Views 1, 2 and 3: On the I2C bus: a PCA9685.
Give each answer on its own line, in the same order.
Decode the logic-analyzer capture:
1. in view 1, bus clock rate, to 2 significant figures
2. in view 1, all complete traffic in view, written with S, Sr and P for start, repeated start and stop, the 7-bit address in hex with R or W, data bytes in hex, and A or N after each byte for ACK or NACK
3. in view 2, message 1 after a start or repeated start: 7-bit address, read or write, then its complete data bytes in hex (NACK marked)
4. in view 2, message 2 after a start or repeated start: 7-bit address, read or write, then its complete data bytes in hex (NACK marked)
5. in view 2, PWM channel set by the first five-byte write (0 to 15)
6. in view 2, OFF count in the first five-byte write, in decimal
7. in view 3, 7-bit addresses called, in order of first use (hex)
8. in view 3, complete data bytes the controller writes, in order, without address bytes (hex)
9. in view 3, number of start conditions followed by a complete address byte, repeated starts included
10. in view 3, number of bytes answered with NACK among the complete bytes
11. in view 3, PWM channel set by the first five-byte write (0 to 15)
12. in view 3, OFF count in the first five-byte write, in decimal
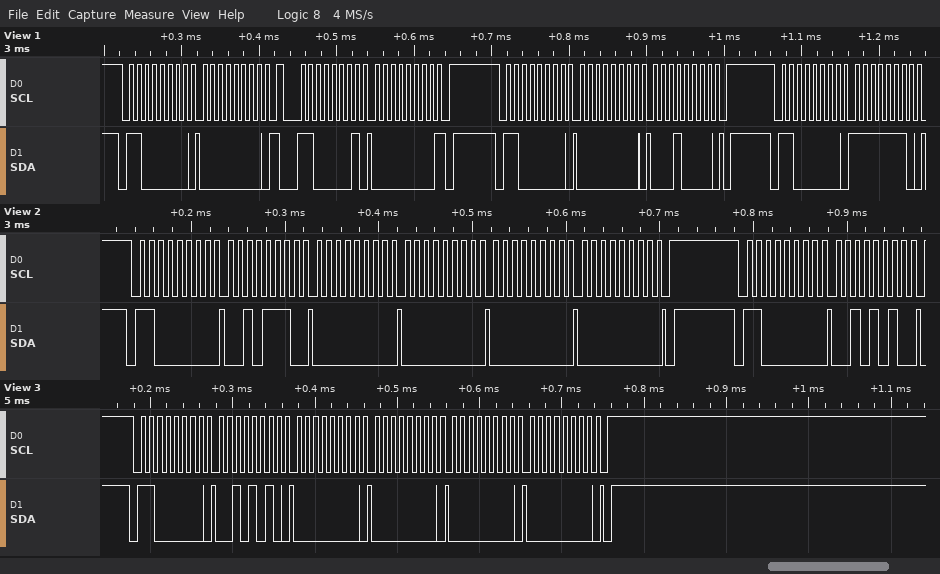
100 kHz
S 60W A 00 A Sr 60R A 00 N P S 60W A 00 A 10 A P S 60W A FE A
0x60 write: 2E 00 00 00 00
0x60 write: 2A
10
0
0x60
2A 00 00 00 00
1
0
9
0
